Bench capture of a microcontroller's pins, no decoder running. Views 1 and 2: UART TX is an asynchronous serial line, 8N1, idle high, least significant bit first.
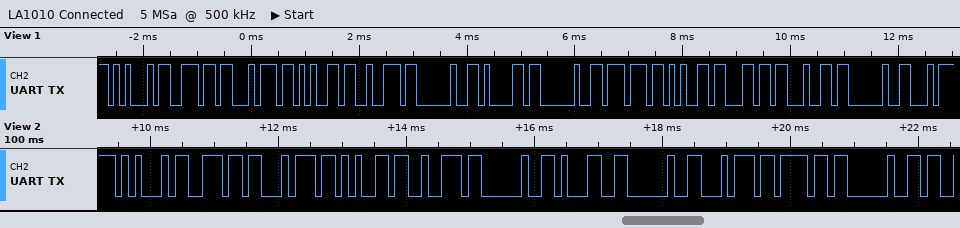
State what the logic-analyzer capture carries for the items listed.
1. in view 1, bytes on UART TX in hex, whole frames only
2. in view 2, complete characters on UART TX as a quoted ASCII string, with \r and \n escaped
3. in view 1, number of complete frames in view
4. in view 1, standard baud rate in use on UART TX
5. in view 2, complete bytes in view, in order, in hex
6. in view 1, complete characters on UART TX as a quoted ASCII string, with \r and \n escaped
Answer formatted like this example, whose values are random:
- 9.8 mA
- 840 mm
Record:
- 0x45 0x6E 0x74 0x65 0x72 0x20 0x61 0x20 0x77 0x65 0x6C 0x64 0x20
- "Enter 1 to "
- 13
- 9600 baud
- 45 6E 74 65 72 20 31 20 74 6F 20
- "Enter a weld "
